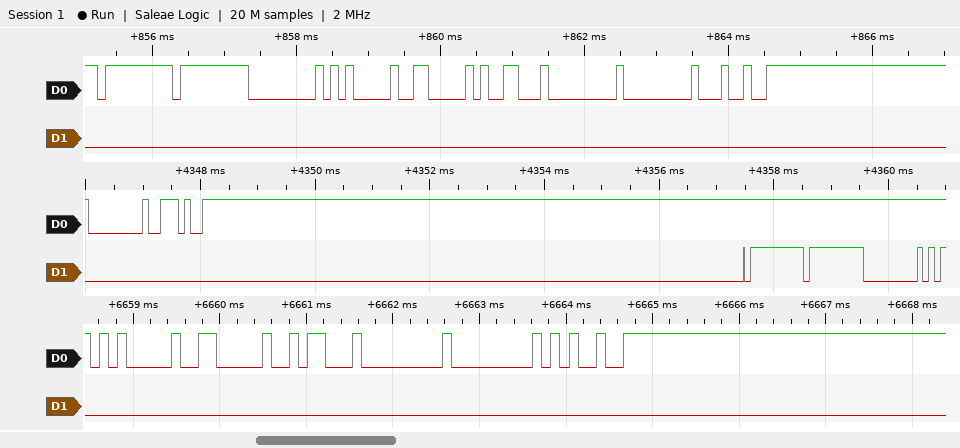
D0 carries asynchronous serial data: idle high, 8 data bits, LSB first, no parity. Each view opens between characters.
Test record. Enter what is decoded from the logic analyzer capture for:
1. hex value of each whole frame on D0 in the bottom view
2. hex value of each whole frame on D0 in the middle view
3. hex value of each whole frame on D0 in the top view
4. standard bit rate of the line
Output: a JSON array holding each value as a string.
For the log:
["05, 06, 1A, 00, 00, 25", "00, 2E", "FF, FF, 00, 05, 06, 19, 00, 00, 24", "9600 baud"]
